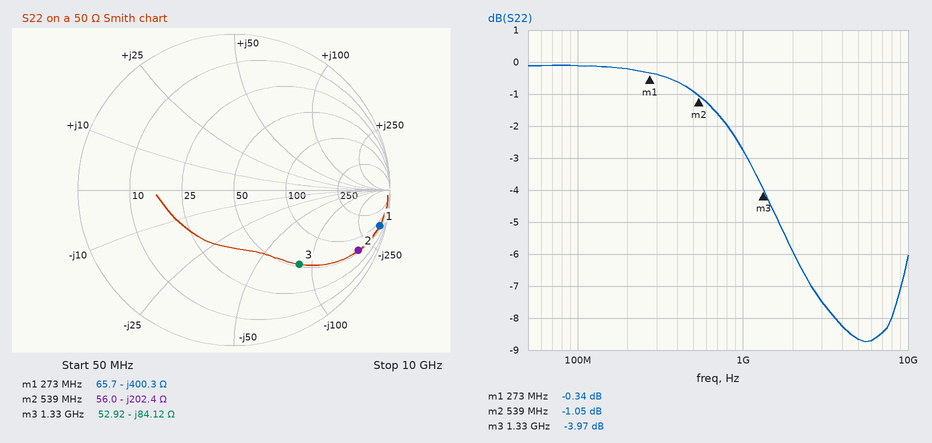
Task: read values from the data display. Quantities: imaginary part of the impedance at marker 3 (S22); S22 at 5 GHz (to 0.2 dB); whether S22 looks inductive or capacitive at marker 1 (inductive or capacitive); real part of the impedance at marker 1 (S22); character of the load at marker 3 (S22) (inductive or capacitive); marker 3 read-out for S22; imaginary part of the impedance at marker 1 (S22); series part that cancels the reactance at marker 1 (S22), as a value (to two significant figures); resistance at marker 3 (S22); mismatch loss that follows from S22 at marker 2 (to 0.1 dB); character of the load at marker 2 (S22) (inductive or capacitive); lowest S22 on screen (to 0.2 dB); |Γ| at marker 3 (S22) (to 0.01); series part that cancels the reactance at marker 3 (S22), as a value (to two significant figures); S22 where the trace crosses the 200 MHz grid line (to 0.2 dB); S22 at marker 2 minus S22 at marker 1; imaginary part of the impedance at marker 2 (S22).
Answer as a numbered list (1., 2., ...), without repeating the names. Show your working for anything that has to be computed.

1. -84.12 Ω
2. -8.6 dB
3. capacitive
4. 65.7 Ω
5. capacitive
6. -3.97 dB
7. -400.3 Ω
8. L = 400.3 Ω/(2π × 273 MHz) ≈ 233 nH, so 230 nH to two significant figures
9. 52.92 Ω
10. −10 log10(1 − 10^(-1.05/10)) ≈ 6.7 dB
11. capacitive
12. -8.8 dB
13. 0.63
14. L = 84.12 Ω/(2π × 1.33 GHz) ≈ 10 nH
15. -0.2 dB
16. -1.05 − (-0.34) = -0.71 dB
17. -202.4 Ω
